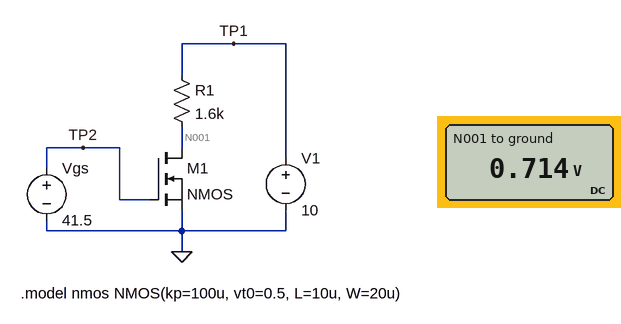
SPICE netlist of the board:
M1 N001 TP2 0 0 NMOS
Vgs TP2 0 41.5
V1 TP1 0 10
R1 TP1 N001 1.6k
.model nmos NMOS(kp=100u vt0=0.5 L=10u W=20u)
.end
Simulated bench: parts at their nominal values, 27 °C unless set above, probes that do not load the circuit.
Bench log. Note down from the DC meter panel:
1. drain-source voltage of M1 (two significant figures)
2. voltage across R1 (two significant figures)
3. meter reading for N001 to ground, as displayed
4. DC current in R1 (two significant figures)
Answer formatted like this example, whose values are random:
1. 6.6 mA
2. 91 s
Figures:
1. 710 mV
2. 9.3 V
3. 0.714 V
4. 5.8 mA
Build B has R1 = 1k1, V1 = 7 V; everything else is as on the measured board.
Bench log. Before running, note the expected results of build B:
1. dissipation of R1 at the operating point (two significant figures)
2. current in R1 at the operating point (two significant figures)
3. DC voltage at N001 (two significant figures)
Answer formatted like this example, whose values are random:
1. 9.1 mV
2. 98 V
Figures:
1. 36 mW
2. 5.7 mA
3. 700 mV
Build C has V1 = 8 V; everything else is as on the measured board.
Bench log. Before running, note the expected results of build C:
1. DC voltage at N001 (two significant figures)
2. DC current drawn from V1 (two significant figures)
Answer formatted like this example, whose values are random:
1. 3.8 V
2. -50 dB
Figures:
1. 570 mV
2. 4.6 mA
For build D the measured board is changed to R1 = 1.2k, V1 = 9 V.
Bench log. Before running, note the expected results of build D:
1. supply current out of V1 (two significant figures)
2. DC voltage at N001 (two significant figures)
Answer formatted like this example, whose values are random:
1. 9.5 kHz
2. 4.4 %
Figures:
1. 6.8 mA
2. 840 mV
